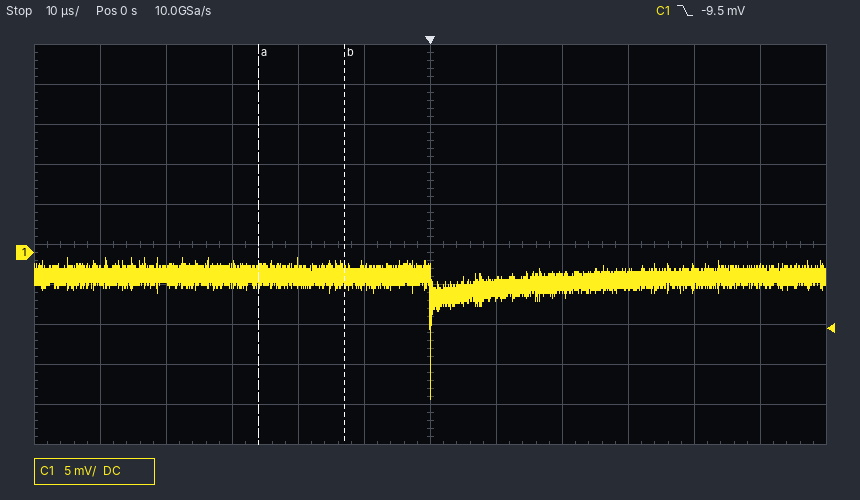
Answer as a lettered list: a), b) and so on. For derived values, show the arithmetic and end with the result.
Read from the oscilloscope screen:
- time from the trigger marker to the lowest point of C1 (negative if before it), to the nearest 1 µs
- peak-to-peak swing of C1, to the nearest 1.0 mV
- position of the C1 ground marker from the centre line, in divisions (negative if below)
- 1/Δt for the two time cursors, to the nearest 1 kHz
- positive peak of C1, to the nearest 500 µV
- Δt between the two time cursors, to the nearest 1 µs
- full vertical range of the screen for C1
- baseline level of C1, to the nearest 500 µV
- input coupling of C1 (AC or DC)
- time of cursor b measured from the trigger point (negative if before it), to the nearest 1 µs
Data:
a) 0 µs
b) 18.0 mV
c) -0.2 div
d) 1 / 13 µs ≈ 77 kHz
e) -500 µV
f) 13 µs
g) 50 mV
h) -3.0 mV
i) DC
j) -13 µs
